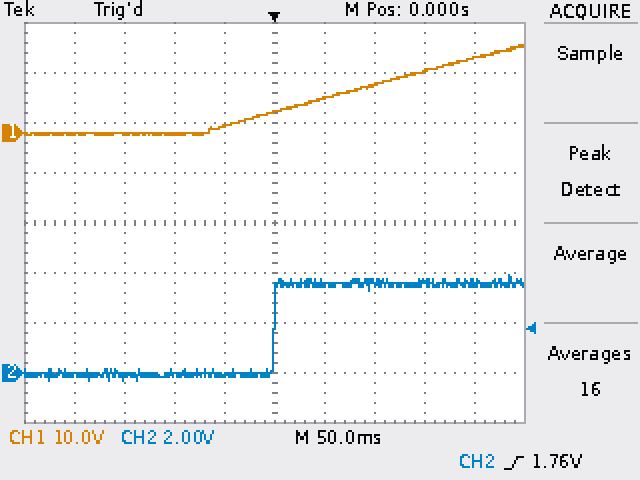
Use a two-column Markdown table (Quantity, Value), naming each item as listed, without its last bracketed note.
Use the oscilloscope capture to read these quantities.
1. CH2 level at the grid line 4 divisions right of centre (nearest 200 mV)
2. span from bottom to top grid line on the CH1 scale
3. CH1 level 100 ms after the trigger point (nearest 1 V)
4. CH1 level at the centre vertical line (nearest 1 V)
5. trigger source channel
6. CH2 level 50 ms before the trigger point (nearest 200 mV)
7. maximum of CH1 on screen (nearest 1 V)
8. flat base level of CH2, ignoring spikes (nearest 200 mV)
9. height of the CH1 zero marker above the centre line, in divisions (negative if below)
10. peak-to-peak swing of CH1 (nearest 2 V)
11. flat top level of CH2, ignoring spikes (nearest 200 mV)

| Quantity | Value |
|---|---|
| CH2 level at the grid line 4 divisions right of centre | 3.6 V |
| span from bottom to top grid line on the CH1 scale | 80 V |
| CH1 level 100 ms after the trigger point | 10 V |
| CH1 level at the centre vertical line | 4 V |
| trigger source channel | CH2 |
| CH2 level 50 ms before the trigger point | 0.0 V |
| maximum of CH1 on screen | 18 V |
| flat base level of CH2, ignoring spikes | 0.0 V |
| height of the CH1 zero marker above the centre line, in divisions | +1.8 div |
| peak-to-peak swing of CH1 | 18 V |
| flat top level of CH2, ignoring spikes | 3.6 V |
